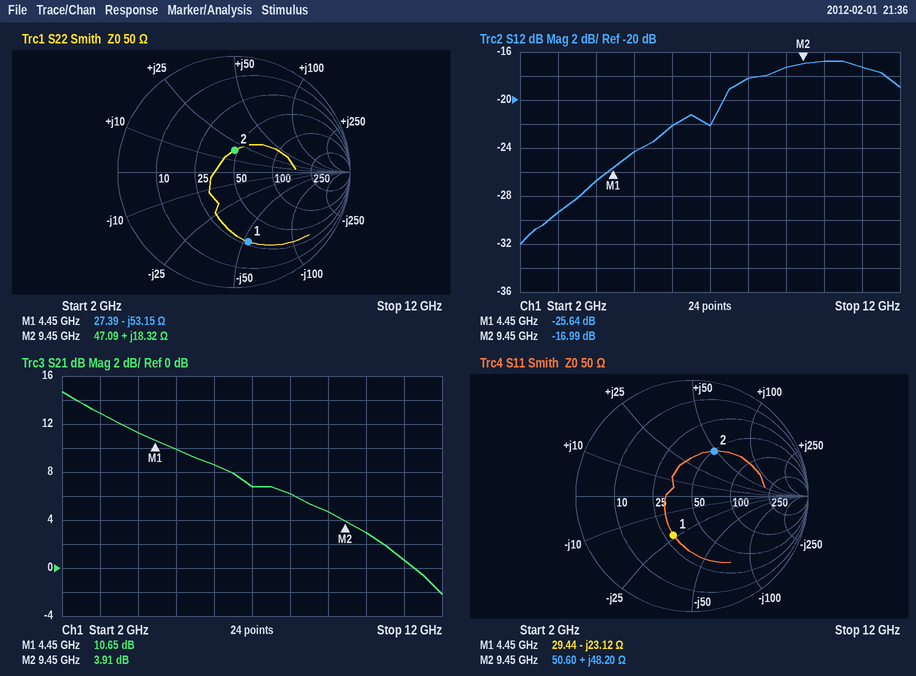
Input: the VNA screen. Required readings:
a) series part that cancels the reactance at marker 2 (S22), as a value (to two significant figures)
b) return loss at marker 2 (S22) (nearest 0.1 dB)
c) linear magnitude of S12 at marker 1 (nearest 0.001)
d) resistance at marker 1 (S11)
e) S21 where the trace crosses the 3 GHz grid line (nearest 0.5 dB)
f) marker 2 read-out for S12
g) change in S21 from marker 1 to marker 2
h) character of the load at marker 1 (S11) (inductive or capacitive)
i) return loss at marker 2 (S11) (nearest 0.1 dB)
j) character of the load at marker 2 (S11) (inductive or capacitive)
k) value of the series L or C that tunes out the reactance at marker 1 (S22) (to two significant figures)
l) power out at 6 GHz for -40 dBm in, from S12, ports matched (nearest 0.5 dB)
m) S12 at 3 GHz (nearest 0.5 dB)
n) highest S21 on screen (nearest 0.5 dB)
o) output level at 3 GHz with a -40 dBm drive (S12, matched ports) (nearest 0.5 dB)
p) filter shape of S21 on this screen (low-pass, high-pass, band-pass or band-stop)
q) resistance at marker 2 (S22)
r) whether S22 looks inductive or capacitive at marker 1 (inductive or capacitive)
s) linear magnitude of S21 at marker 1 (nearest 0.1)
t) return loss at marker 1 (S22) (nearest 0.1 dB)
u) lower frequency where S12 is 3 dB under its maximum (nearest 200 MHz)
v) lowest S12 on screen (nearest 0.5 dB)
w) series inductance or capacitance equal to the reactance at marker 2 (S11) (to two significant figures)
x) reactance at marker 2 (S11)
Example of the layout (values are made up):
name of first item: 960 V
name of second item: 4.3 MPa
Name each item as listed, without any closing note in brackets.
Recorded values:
series part that cancels the reactance at marker 2 (S22), as a value: 920 fF
return loss at marker 2 (S22): 14.5 dB
linear magnitude of S12 at marker 1: 0.052
resistance at marker 1: 29.44 Ω
S21 where the trace crosses the 3 GHz grid line: 13.0 dB
marker 2 read-out for S12: -16.99 dB
change in S21 from marker 1 to marker 2: -6.74 dB
character of the load at marker 1 (S11): capacitive
return loss at marker 2 (S11): 7.3 dB
character of the load at marker 2 (S11): inductive
value of the series L or C that tunes out the reactance at marker 1 (S22): 1.9 nH
power out at 6 GHz for -40 dBm in, from S12, ports matched: -62.0 dBm
S12 at 3 GHz: -29.5 dB
highest S21 on screen: 14.5 dB
output level at 3 GHz with a -40 dBm drive (S12, matched ports): -69.5 dBm
filter shape of S21 on this screen: low-pass
resistance at marker 2: 47.09 Ω
whether S22 looks inductive or capacitive at marker 1: capacitive
linear magnitude of S21 at marker 1: 3.4
return loss at marker 1 (S22): 4.2 dB
lower frequency where S12 is 3 dB under its maximum: 7.4 GHz
lowest S12 on screen: -32.0 dB
series inductance or capacitance equal to the reactance at marker 2 (S11): 810 pH
reactance at marker 2: +48.20 Ω
